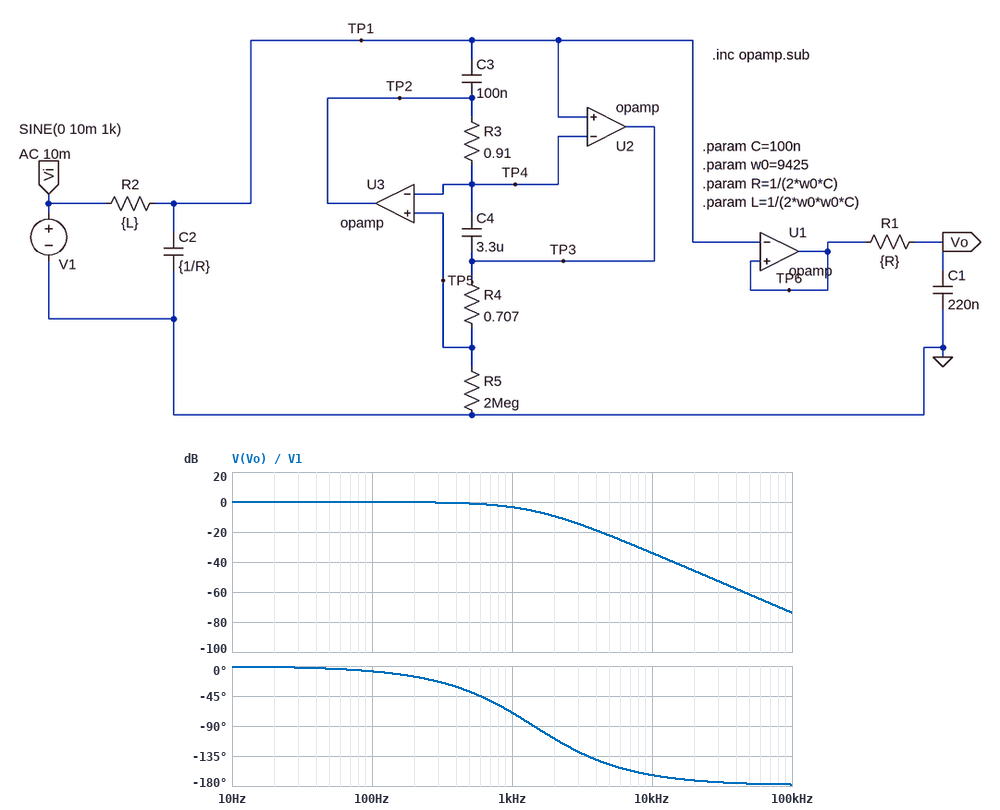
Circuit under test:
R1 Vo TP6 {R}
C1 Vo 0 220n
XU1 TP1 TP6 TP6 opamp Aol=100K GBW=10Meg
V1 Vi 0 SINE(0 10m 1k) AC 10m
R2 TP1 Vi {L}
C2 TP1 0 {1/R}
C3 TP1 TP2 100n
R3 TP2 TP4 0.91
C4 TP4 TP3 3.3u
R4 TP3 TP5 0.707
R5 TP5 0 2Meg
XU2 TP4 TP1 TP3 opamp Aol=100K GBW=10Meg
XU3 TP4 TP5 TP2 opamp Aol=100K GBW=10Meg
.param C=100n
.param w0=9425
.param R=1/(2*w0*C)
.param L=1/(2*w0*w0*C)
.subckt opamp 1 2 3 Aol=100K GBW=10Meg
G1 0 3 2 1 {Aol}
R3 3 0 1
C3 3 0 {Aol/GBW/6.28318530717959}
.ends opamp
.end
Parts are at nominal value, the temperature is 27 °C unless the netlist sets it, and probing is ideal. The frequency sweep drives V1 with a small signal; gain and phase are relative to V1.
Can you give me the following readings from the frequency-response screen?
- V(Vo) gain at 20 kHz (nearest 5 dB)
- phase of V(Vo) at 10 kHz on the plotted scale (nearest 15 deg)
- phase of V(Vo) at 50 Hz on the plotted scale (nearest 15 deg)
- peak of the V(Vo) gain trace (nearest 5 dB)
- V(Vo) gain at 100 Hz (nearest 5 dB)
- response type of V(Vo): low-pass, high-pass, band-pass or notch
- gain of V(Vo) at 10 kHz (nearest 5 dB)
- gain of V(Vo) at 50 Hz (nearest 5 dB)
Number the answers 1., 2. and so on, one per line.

1. -45 dB
2. -165 deg
3. 0 deg
4. 0 dB
5. 0 dB
6. low-pass
7. -35 dB
8. 0 dB
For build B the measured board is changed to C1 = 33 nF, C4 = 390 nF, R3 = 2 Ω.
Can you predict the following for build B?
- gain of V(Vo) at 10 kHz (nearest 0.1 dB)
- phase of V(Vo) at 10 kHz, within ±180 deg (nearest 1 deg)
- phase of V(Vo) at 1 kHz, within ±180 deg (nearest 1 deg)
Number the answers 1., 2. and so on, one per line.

1. -20.0 dB
2. -129 deg
3. -40 deg
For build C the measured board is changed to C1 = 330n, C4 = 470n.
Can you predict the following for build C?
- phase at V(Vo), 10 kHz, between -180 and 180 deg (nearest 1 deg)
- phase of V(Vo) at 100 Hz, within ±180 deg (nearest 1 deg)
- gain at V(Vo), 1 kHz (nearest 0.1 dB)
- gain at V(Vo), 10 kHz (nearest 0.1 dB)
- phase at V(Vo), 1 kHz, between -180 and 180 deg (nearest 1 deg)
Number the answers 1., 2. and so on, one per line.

1. -166 deg
2. -10 deg
3. -5.0 dB
4. -37.4 dB
5. -81 deg
